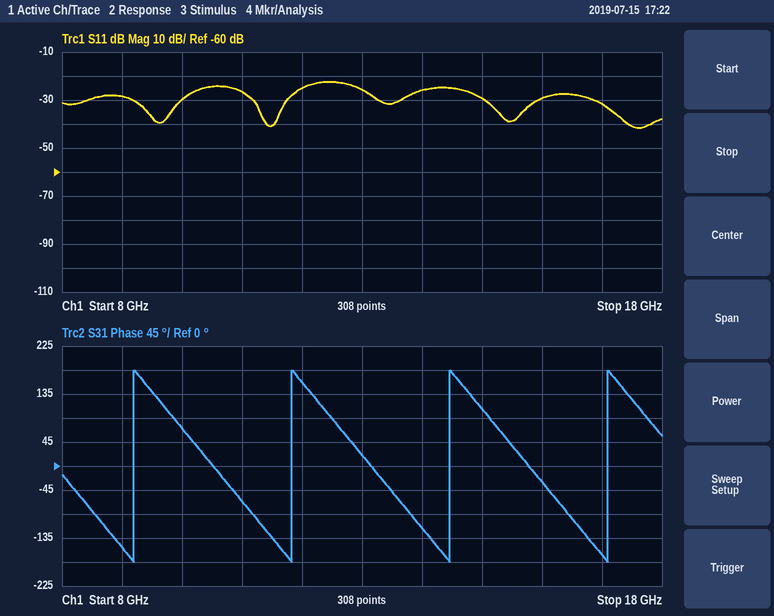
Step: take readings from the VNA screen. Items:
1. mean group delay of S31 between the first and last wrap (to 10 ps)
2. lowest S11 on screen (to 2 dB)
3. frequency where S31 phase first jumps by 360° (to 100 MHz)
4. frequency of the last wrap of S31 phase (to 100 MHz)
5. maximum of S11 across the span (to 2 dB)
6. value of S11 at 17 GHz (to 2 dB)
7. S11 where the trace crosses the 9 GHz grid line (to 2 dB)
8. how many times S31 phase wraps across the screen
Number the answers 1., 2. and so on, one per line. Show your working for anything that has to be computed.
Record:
1. 3 cycles / (17.1 GHz − 9.2 GHz) ≈ 380 ps
2. -42 dB
3. 9.2 GHz
4. 17.1 GHz
5. -22 dB
6. -32 dB
7. -28 dB
8. 4
